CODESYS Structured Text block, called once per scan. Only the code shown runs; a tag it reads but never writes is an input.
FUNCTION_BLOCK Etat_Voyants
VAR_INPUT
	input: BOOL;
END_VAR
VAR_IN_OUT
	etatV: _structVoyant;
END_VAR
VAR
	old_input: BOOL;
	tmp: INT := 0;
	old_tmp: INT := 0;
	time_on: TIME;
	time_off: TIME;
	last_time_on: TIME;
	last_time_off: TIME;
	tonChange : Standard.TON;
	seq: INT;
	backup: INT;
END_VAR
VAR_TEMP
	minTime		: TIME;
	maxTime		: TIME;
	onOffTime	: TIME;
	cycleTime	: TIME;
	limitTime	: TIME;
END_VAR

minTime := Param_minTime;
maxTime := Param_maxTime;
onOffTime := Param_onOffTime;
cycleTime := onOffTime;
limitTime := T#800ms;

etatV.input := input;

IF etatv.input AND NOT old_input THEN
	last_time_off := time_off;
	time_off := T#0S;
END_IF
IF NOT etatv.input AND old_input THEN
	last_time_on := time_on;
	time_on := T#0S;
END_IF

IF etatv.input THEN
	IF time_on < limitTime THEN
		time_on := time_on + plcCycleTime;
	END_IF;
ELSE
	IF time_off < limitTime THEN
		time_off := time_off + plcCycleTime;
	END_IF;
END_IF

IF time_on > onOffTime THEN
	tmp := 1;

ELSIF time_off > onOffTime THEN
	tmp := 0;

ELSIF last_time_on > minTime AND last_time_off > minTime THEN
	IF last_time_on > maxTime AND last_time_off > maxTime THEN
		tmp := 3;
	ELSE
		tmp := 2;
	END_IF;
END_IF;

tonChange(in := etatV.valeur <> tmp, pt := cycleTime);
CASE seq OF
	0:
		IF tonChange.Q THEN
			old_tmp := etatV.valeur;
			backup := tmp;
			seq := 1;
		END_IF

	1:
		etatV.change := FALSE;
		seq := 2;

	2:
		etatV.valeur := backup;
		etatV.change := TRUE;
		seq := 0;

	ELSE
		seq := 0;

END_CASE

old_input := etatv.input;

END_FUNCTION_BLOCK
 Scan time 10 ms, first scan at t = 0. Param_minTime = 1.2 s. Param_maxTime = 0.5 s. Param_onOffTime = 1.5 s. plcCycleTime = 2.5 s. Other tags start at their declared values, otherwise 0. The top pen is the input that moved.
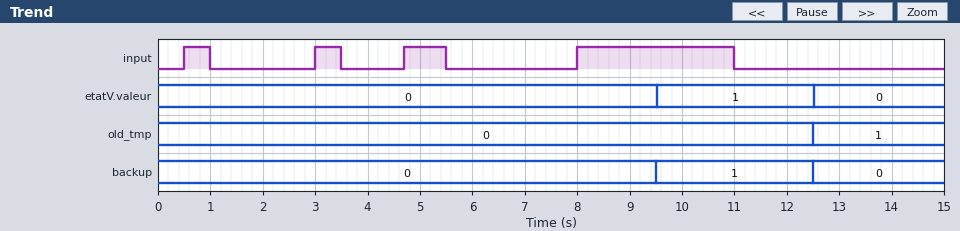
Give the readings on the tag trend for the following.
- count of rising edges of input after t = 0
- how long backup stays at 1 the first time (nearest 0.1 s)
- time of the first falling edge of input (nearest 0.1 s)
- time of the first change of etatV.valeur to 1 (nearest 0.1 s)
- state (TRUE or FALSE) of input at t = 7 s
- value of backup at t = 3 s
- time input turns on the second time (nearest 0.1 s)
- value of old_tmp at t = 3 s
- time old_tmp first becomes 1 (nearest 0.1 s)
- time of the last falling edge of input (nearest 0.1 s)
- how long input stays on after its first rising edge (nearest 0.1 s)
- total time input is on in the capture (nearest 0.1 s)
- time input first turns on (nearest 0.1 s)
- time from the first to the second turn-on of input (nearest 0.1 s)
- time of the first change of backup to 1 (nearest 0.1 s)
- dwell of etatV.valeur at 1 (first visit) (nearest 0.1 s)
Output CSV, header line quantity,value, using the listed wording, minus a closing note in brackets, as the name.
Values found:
quantity,value
count of rising edges of input after t = 0,4
how long backup stays at 1 the first time,3.0 s
time of the first falling edge of input,1.0 s
time of the first change of etatV.valeur to 1,9.5 s
state (TRUE or FALSE) of input at t = 7 s,FALSE
value of backup at t = 3 s,0
time input turns on the second time,3.0 s
value of old_tmp at t = 3 s,0
time old_tmp first becomes 1,12.5 s
time of the last falling edge of input,11.0 s
how long input stays on after its first rising edge,0.5 s
total time input is on in the capture,4.8 s
time input first turns on,0.5 s
time from the first to the second turn-on of input,2.5 s
time of the first change of backup to 1,9.5 s
dwell of etatV.valeur at 1 (first visit),3.0 s
